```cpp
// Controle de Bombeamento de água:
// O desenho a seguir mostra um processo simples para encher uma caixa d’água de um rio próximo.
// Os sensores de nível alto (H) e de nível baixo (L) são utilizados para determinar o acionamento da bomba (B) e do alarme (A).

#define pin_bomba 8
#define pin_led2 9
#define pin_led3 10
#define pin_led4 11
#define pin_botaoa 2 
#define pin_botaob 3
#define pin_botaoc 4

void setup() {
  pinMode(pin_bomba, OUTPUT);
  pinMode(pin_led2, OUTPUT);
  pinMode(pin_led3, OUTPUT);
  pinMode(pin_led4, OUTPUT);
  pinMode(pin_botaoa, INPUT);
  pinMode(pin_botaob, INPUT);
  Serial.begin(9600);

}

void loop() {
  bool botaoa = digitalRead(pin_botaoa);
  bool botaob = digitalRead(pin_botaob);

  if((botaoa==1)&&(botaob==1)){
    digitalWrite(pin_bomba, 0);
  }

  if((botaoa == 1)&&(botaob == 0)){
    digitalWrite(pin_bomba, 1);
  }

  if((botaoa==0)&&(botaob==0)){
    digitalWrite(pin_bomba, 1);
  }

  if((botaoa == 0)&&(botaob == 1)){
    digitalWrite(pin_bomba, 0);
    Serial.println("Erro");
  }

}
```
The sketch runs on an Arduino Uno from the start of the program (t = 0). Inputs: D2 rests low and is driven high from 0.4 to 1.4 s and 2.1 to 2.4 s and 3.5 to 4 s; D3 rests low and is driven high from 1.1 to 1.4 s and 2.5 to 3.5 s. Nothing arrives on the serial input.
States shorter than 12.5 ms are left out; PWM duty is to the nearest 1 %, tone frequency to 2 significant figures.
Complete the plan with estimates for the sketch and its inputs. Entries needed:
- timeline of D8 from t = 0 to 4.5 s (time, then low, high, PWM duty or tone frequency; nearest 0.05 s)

0 s high; 1.1 s low; 1.4 s high; 2.5 s low; 3.5 s high
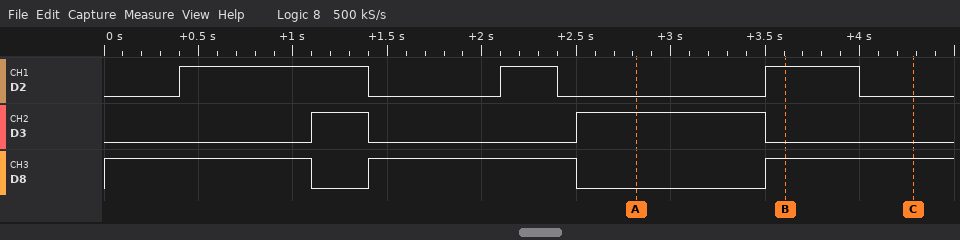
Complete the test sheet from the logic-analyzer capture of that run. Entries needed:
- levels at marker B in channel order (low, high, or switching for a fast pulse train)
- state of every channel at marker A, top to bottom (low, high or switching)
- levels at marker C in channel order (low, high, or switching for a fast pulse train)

D2 high, D3 low, D8 high
D2 low, D3 high, D8 low
D2 low, D3 low, D8 high
